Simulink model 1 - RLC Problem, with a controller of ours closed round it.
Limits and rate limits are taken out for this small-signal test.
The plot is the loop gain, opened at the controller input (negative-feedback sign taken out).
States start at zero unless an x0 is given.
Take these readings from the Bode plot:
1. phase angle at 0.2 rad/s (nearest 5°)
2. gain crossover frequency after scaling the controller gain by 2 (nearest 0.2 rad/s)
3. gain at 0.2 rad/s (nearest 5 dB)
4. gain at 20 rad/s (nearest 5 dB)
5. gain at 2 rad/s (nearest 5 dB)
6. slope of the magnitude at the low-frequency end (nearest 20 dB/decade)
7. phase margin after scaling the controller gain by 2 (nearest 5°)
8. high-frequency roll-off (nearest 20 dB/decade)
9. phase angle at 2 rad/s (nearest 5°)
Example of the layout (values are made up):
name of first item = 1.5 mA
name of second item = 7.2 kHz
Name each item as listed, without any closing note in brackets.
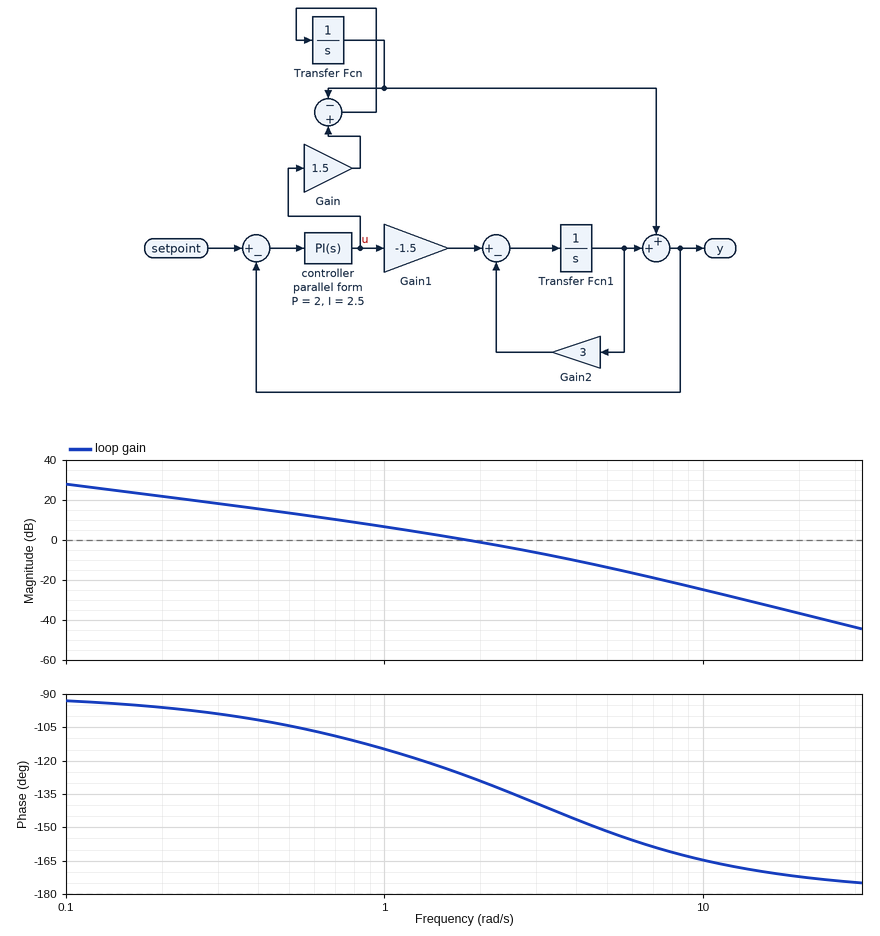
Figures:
phase angle at 0.2 rad/s = -95°
gain crossover frequency after scaling the controller gain by 2 = 3.0 rad/s
gain at 0.2 rad/s = 20 dB
gain at 20 rad/s = -35 dB
gain at 2 rad/s = 0 dB
slope of the magnitude at the low-frequency end = -20 dB/decade
phase margin after scaling the controller gain by 2 = 40°
high-frequency roll-off = -40 dB/decade
phase angle at 2 rad/s = -130°
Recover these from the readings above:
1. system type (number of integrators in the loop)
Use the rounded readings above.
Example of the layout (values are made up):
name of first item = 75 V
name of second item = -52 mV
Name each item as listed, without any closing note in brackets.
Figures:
system type = 1
